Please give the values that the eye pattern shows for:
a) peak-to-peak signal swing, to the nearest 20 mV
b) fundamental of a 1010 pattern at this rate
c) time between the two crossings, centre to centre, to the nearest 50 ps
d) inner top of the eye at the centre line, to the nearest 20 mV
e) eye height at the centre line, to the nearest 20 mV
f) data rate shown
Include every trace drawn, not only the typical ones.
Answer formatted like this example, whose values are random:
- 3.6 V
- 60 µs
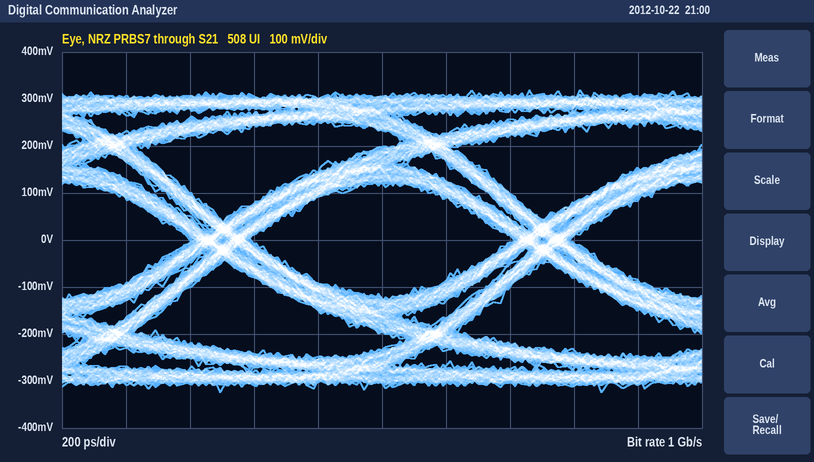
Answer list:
- 640 mV
- 500 MHz
- 1.00 ns
- 120 mV
- 240 mV
- 1 Gb/s
